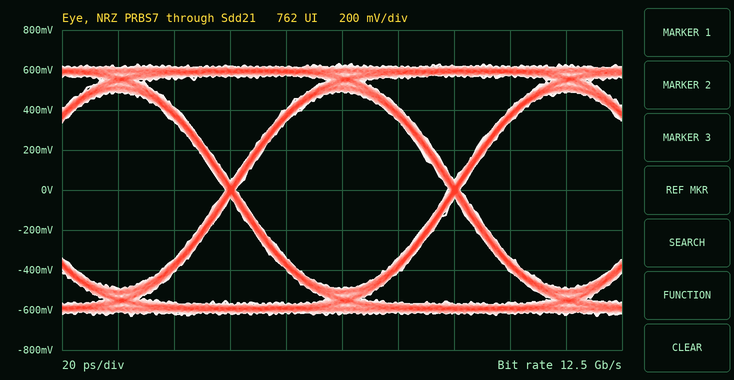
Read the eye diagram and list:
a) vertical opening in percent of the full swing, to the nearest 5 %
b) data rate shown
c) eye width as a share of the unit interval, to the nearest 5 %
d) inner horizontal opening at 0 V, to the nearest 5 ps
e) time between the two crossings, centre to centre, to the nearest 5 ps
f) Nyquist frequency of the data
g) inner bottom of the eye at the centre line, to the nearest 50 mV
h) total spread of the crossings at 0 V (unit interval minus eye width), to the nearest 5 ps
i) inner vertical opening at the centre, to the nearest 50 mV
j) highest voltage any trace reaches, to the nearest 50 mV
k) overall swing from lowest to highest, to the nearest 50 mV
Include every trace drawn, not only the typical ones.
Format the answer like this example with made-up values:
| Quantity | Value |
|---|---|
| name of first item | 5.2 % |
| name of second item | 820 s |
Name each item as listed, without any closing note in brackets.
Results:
| Quantity | Value |
|---|---|
| vertical opening in percent of the full swing, to the nearest 5 % | 80 % |
| data rate shown | 12.5 Gb/s |
| eye width as a share of the unit interval, to the nearest 5 % | 95 % |
| inner horizontal opening at 0 V, to the nearest 5 ps | 75 ps |
| time between the two crossings, centre to centre, to the nearest 5 ps | 80 ps |
| Nyquist frequency of the data | 6.25 GHz |
| inner bottom of the eye at the centre line, to the nearest 50 mV | -500 mV |
| total spread of the crossings at 0 V (unit interval minus eye width), to the nearest 5 ps | 5 ps |
| inner vertical opening at the centre, to the nearest 50 mV | 1.00 V |
| highest voltage any trace reaches, to the nearest 50 mV | 650 mV |
| overall swing from lowest to highest, to the nearest 50 mV | 1.25 V |
